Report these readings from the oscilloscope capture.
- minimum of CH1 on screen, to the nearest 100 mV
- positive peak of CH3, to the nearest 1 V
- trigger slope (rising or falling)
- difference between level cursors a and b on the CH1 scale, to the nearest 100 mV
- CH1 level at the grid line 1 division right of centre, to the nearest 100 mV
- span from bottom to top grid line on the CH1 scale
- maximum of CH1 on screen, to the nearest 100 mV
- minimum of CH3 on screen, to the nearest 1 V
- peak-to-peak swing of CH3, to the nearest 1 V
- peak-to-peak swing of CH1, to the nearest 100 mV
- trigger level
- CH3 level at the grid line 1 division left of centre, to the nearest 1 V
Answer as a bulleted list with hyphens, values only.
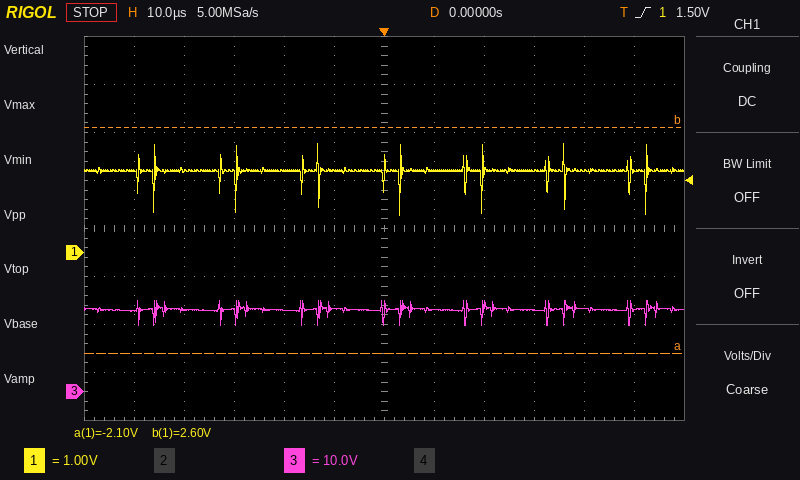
- 800 mV
- 19 V
- rising
- 4.7 V
- 1.7 V
- 8 V
- 2.3 V
- 14 V
- 5 V
- 1.5 V
- 1.50 V
- 17 V
